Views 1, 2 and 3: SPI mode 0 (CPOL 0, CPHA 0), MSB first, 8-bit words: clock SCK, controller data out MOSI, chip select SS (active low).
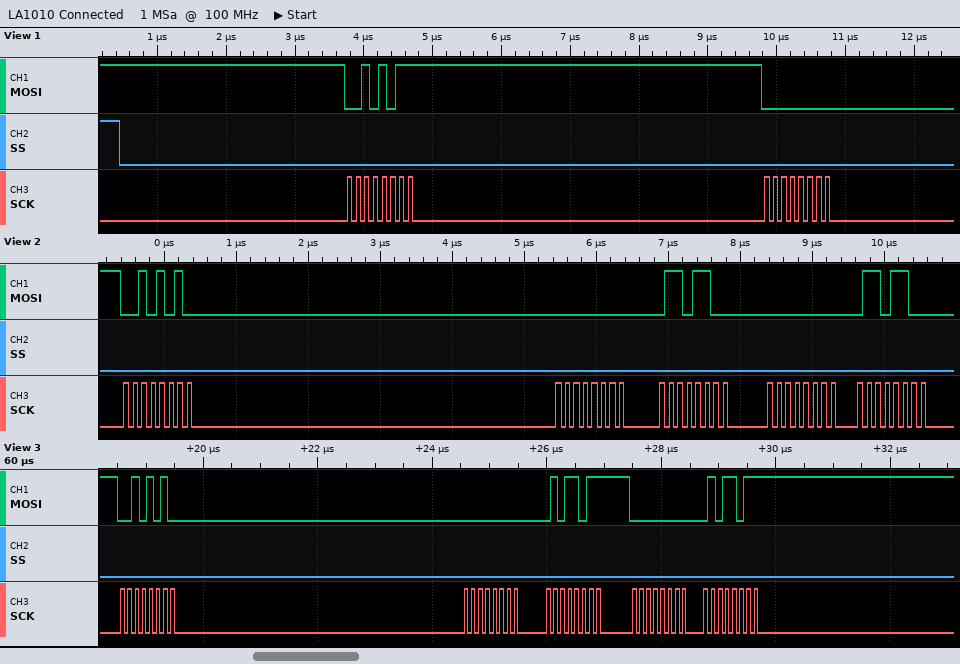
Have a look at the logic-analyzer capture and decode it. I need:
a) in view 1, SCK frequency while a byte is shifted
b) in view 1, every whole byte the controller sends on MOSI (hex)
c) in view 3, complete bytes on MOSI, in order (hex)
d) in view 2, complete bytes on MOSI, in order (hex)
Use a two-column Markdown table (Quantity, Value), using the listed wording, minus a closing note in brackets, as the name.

| Quantity | Value |
|---|---|
| in view 1, SCK frequency while a byte is shifted | 8 MHz |
| in view 1, every whole byte the controller sends on MOSI | 2B 00 |
| in view 3, complete bytes on MOSI, in order | 2A 00 5B 00 5B |
| in view 2, complete bytes on MOSI, in order | 2A 00 6C 00 6C |
